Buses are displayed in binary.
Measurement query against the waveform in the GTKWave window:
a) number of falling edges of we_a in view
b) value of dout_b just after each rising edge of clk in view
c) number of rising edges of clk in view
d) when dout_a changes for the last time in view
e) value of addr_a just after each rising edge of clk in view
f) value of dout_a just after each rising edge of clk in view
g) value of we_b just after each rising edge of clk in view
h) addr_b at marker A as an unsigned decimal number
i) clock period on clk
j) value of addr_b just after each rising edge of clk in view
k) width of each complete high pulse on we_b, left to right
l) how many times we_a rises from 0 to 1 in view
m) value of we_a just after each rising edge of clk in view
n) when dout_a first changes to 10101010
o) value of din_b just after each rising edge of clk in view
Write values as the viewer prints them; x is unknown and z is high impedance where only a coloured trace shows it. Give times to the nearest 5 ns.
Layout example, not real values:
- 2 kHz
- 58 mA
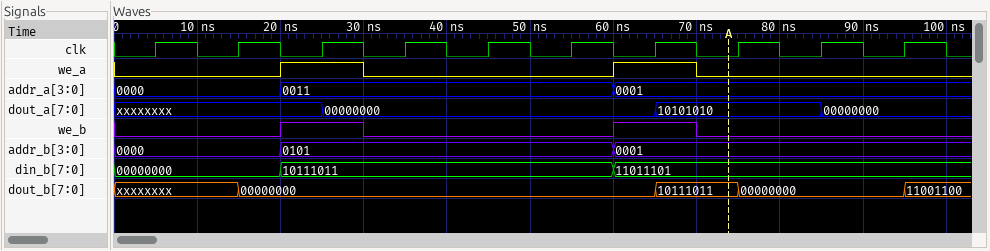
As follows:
- 2
- xxxxxxxx, 00000000, 00000000, 00000000, 00000000, 00000000, 10111011, 00000000, 00000000, 11001100
- 10
- 85 ns
- 0000, 0000, 0011, 0011, 0011, 0011, 0001, 0001, 0001, 0001
- xxxxxxxx, xxxxxxxx, 00000000, 00000000, 00000000, 00000000, 10101010, 10101010, 00000000, 00000000
- 0 0 1 0 0 0 1 0 0 0
- 1
- 10 ns
- 0000, 0000, 0101, 0101, 0101, 0101, 0001, 0001, 0001, 0001
- 10 ns, 10 ns
- 2
- 0 0 1 0 0 0 1 0 0 0
- 65 ns
- 00000000, 00000000, 10111011, 10111011, 10111011, 10111011, 11011101, 11011101, 11011101, 11011101
